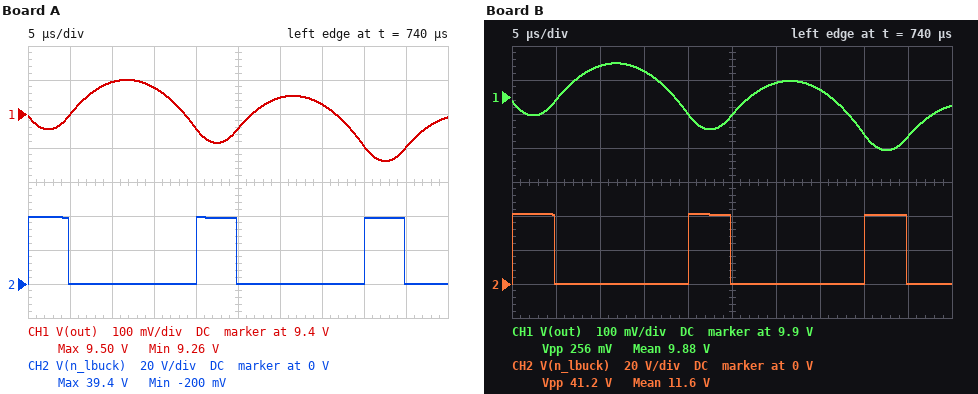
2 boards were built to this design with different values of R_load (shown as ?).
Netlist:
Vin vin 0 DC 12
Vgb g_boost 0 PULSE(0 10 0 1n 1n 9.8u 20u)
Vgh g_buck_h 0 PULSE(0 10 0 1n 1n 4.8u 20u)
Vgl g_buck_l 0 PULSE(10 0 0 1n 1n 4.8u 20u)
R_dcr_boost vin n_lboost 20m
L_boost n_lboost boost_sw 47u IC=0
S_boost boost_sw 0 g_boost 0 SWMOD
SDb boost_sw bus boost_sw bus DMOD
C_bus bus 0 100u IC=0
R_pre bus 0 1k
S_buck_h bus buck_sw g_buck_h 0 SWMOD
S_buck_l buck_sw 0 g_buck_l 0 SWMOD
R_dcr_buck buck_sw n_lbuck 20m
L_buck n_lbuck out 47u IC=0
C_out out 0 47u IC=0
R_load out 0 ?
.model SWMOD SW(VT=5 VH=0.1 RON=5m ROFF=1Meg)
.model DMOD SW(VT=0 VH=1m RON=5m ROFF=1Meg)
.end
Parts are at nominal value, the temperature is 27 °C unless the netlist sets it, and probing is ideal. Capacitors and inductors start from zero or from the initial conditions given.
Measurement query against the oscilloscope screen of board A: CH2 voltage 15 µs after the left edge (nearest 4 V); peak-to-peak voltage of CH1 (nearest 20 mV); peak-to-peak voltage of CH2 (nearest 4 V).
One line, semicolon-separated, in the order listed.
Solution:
0 V; 240 mV; 40 V
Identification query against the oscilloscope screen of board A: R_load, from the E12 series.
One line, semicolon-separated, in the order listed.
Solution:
1.8 Ω
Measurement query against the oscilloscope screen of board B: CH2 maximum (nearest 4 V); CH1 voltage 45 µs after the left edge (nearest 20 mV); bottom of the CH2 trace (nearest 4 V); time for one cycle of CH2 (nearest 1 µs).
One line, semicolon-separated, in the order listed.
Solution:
40 V; 9.78 V; 0 V; 20 µs
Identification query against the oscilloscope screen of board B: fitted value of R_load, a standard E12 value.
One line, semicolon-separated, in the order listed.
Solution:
2.7 Ω
